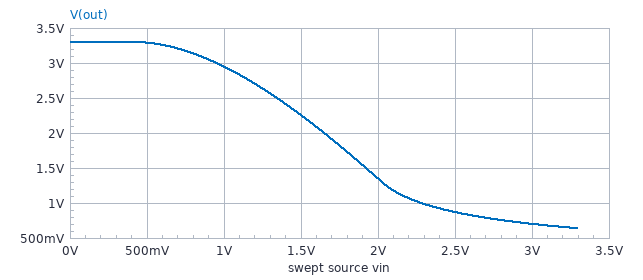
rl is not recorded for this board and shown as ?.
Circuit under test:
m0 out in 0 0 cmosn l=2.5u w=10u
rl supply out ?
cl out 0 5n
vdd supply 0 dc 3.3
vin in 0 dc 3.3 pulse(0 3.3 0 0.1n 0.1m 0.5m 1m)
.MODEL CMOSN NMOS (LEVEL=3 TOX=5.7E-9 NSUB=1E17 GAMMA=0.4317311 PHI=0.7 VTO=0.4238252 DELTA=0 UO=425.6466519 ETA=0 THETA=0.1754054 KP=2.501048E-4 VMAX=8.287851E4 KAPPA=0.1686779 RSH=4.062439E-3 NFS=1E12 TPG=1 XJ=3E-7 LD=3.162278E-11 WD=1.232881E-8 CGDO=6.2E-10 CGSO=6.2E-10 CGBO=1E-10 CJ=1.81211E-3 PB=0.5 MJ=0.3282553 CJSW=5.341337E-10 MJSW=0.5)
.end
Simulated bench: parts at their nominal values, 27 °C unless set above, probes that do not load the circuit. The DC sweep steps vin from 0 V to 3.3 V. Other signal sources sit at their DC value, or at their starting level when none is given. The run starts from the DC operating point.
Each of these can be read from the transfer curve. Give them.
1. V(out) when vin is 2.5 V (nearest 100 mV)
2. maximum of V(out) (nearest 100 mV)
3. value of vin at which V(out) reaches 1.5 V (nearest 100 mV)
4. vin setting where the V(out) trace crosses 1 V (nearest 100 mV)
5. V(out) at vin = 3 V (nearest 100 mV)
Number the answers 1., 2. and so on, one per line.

1. 900 mV
2. 3.3 V
3. 1.9 V
4. 2.3 V
5. 700 mV
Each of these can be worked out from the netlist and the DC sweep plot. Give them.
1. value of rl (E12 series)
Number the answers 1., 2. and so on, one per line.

1. 2.7 kΩ
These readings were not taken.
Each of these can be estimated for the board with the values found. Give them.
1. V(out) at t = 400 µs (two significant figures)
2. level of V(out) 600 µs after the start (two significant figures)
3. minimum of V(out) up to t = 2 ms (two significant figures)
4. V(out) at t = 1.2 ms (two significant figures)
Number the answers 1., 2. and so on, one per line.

1. 640 mV
2. 3.2 V
3. 640 mV
4. 640 mV
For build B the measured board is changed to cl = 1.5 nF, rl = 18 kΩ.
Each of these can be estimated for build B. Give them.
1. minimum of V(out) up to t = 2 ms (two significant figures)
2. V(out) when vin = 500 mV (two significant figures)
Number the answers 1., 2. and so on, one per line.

1. 96 mV
2. 3.2 V
